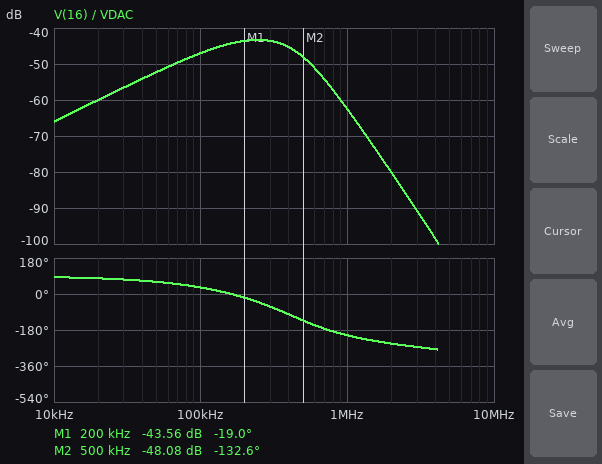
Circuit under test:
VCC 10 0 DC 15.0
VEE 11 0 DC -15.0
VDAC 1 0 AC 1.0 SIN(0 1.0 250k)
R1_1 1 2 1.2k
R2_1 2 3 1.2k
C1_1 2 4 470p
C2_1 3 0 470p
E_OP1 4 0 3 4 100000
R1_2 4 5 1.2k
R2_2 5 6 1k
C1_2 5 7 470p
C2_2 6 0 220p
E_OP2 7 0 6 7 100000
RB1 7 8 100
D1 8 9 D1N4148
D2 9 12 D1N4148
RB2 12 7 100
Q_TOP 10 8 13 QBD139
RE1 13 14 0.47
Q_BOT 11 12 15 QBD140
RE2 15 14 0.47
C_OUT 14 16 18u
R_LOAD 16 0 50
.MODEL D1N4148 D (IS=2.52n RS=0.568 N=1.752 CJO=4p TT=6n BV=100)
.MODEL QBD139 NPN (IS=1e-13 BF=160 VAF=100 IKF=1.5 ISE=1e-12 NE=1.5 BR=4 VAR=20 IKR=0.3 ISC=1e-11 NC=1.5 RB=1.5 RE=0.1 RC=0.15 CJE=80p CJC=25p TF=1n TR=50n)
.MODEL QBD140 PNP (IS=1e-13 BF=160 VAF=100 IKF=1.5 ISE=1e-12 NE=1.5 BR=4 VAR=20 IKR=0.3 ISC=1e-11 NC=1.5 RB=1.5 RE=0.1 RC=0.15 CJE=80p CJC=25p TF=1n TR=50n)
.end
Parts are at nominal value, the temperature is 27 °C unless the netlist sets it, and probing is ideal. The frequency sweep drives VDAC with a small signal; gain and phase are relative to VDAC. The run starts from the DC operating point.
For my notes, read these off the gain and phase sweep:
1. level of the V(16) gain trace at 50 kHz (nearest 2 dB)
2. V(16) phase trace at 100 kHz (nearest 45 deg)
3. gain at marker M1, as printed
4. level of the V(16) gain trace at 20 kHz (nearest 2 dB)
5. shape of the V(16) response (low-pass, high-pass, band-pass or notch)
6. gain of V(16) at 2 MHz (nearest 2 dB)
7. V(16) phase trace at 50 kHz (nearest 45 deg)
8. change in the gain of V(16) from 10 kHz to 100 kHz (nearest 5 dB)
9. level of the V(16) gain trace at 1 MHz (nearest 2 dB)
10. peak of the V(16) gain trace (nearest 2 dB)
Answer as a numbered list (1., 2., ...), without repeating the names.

1. -52 dB
2. 45 deg
3. -43.56 dB
4. -60 dB
5. band-pass
6. -80 dB
7. 45 deg
8. 20 dB
9. -62 dB
10. -44 dB
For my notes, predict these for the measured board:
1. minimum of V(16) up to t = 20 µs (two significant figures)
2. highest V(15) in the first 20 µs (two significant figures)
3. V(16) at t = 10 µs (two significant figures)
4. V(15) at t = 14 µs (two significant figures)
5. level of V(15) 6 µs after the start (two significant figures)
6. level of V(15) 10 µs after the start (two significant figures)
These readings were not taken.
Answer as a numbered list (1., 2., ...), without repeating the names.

1. -7.0 mV
2. 32 mV
3. 5.0 mV
4. 5.0 mV
5. 5.0 mV
6. 5.0 mV
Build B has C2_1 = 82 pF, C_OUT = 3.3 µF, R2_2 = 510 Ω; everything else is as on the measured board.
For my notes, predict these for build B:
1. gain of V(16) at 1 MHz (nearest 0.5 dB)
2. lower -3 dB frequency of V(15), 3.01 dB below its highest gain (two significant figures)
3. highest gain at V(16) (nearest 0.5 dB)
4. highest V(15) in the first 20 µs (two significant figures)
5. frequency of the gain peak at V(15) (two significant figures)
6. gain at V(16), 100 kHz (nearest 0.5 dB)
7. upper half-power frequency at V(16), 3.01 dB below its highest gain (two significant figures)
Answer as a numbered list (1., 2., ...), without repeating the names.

1. -39.5 dB
2. 360 kHz
3. -31.0 dB
4. 400 mV
5. 570 kHz
6. -46.0 dB
7. 790 kHz
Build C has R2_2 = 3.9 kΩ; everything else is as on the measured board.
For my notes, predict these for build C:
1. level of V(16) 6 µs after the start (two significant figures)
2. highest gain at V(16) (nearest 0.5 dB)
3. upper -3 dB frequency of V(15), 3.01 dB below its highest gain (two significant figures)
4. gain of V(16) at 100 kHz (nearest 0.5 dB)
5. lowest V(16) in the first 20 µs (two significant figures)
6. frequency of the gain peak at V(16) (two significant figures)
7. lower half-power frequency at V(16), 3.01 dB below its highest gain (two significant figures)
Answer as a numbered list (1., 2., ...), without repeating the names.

1. 4.0 mV
2. -46.0 dB
3. 280 kHz
4. -47.5 dB
5. -4.4 mV
6. 160 kHz
7. 77 kHz
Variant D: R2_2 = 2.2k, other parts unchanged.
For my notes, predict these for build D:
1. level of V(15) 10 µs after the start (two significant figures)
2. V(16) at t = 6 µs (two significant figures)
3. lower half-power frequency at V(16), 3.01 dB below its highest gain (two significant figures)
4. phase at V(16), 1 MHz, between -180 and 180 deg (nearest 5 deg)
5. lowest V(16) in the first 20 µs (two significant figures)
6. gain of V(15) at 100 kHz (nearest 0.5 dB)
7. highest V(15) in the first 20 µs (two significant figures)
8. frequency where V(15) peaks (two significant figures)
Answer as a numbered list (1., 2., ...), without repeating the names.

1. 5.5 mV
2. 5.4 mV
3. 96 kHz
4. 140 deg
5. -6.0 mV
6. -47.0 dB
7. 7.1 mV
8. 200 kHz
